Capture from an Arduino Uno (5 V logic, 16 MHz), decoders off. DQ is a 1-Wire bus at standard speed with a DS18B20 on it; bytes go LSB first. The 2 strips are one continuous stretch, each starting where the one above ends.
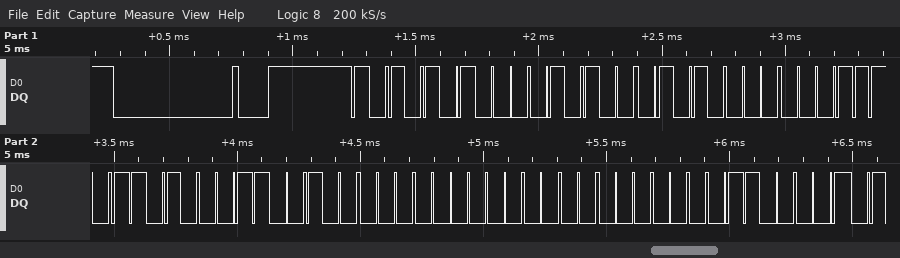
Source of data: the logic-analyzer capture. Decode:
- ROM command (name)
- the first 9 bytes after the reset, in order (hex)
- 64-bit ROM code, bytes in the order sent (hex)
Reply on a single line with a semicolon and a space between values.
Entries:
Match ROM; 55 28 0A B8 C5 04 00 00 86; 28 0A B8 C5 04 00 00 86
